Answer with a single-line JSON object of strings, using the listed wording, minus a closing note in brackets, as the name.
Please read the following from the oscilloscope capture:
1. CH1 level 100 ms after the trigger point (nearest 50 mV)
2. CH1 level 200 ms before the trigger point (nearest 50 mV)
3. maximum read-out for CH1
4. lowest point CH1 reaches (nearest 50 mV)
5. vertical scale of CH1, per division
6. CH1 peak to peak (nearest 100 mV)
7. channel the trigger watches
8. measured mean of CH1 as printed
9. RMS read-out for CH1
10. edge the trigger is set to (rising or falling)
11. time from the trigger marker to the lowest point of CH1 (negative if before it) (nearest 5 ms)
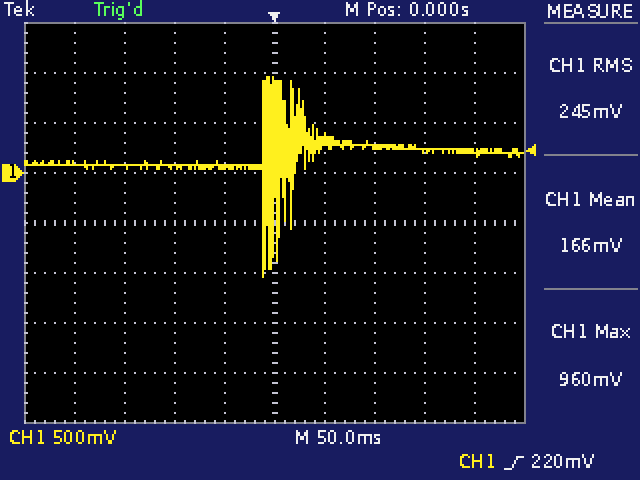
{"CH1 level 100 ms after the trigger point": "250 mV", "CH1 level 200 ms before the trigger point": "100 mV", "maximum read-out for CH1": "960 mV", "lowest point CH1 reaches": "-1.05 V", "vertical scale of CH1, per division": "500 mV", "CH1 peak to peak": "2.00 V", "channel the trigger watches": "CH1", "measured mean of CH1 as printed": "166 mV", "RMS read-out for CH1": "245 mV", "edge the trigger is set to": "rising", "time from the trigger marker to the lowest point of CH1 (negative if before it)": "-10 ms"}
